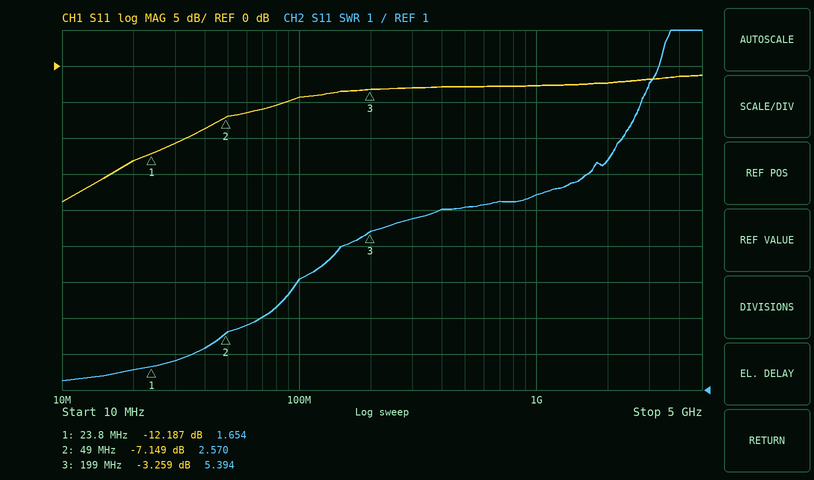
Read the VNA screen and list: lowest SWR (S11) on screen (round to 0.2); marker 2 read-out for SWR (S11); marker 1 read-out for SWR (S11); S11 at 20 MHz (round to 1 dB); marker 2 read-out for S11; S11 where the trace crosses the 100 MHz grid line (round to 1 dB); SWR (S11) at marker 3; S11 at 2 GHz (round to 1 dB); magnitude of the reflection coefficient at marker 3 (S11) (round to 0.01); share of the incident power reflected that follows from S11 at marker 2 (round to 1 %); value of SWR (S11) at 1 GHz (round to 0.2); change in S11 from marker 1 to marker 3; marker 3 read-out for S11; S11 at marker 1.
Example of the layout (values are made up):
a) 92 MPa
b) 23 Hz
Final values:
a) 1.2
b) 2.570
c) 1.654
d) -13 dB
e) -7.149 dB
f) -4 dB
g) 5.394
h) -2 dB
i) 0.69
j) 19 %
k) 6.4
l) 8.928 dB
m) -3.259 dB
n) -12.187 dB
